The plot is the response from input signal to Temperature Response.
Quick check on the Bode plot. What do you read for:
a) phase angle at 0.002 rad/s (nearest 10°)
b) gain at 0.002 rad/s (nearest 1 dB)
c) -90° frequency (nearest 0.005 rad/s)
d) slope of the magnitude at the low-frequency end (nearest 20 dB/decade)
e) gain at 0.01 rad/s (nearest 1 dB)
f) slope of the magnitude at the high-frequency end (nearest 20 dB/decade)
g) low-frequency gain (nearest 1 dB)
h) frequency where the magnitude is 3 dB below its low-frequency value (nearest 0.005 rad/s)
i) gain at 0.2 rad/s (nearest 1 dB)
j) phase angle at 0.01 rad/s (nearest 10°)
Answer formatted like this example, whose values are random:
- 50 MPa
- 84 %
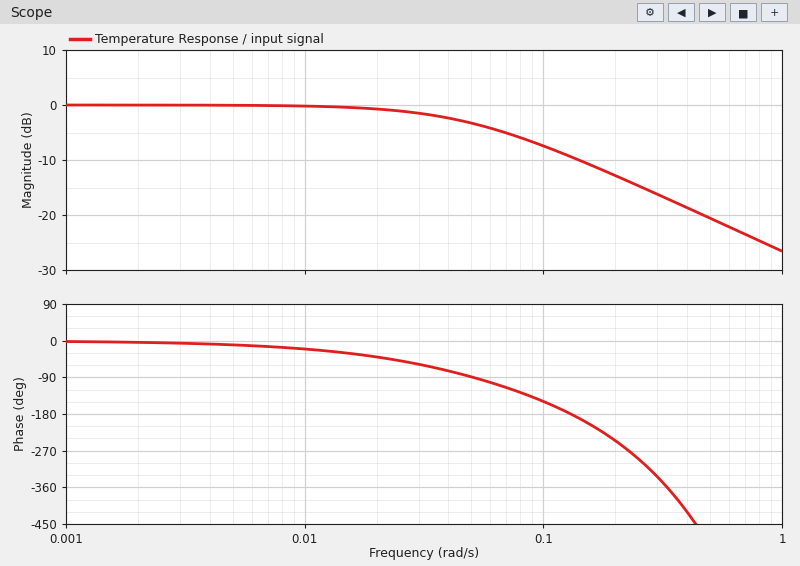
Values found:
- 0°
- 0 dB
- 0.050 rad/s
- 0 dB/decade
- 0 dB
- -20 dB/decade
- 0 dB
- 0.045 rad/s
- -13 dB
- -20°
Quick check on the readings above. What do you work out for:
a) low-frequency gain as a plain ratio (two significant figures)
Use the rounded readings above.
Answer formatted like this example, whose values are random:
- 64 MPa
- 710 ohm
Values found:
- 1.0
